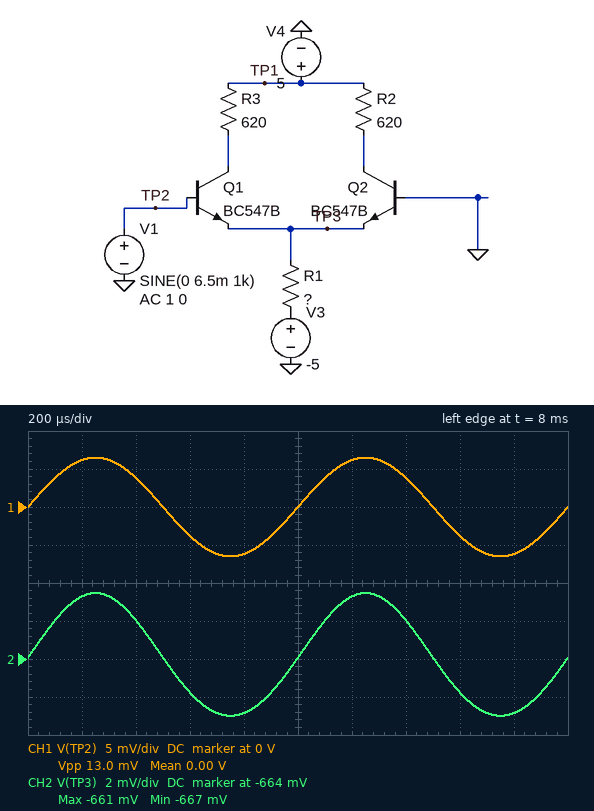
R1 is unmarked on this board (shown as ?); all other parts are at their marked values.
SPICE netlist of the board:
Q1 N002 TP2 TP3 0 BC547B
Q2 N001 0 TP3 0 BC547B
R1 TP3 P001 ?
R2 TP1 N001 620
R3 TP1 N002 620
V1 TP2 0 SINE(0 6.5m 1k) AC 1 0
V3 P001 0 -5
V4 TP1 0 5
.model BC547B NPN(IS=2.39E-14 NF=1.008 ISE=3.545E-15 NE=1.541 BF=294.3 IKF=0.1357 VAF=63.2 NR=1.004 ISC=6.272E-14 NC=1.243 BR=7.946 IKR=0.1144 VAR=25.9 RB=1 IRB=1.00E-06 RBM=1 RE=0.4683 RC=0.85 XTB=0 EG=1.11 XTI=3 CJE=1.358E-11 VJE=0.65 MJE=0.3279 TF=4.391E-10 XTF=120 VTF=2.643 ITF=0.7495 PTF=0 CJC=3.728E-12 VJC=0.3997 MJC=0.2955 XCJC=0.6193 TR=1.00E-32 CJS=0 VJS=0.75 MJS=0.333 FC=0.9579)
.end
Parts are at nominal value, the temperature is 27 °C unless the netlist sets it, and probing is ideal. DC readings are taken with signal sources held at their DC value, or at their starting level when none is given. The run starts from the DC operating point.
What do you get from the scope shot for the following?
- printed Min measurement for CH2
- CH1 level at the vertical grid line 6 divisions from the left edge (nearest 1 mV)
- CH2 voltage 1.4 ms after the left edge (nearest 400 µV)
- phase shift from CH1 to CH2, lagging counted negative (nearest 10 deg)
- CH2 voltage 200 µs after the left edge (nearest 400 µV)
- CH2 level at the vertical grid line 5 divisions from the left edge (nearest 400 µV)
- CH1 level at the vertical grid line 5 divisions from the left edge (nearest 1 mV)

-667 mV
6 mV
-662.0 mV
0 deg
-660.8 mV
-664.0 mV
0 V
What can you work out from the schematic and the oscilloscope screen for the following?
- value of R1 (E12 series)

820 Ω
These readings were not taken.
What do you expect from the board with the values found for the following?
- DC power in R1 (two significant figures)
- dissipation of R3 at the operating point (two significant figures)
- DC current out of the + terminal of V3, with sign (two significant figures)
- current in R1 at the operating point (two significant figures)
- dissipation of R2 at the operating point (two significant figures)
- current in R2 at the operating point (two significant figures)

23 mW
4.3 mW
-5.3 mA
5.3 mA
4.3 mW
2.6 mA
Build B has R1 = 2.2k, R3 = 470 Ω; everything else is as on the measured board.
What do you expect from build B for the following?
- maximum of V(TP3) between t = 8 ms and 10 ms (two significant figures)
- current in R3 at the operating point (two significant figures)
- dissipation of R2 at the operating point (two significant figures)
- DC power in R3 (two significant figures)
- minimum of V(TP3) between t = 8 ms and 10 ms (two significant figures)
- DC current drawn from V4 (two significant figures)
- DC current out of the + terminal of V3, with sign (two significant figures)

-630 mV
990 µA
600 µW
460 µW
-640 mV
2.0 mA
-2.0 mA
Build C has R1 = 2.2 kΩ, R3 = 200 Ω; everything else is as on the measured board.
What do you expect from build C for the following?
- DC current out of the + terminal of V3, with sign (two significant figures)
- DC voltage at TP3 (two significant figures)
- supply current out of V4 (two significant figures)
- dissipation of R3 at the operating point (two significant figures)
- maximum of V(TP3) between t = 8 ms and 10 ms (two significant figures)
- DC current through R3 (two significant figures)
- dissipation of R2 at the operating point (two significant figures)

-2.0 mA
-640 mV
2.0 mA
200 µW
-630 mV
990 µA
600 µW
